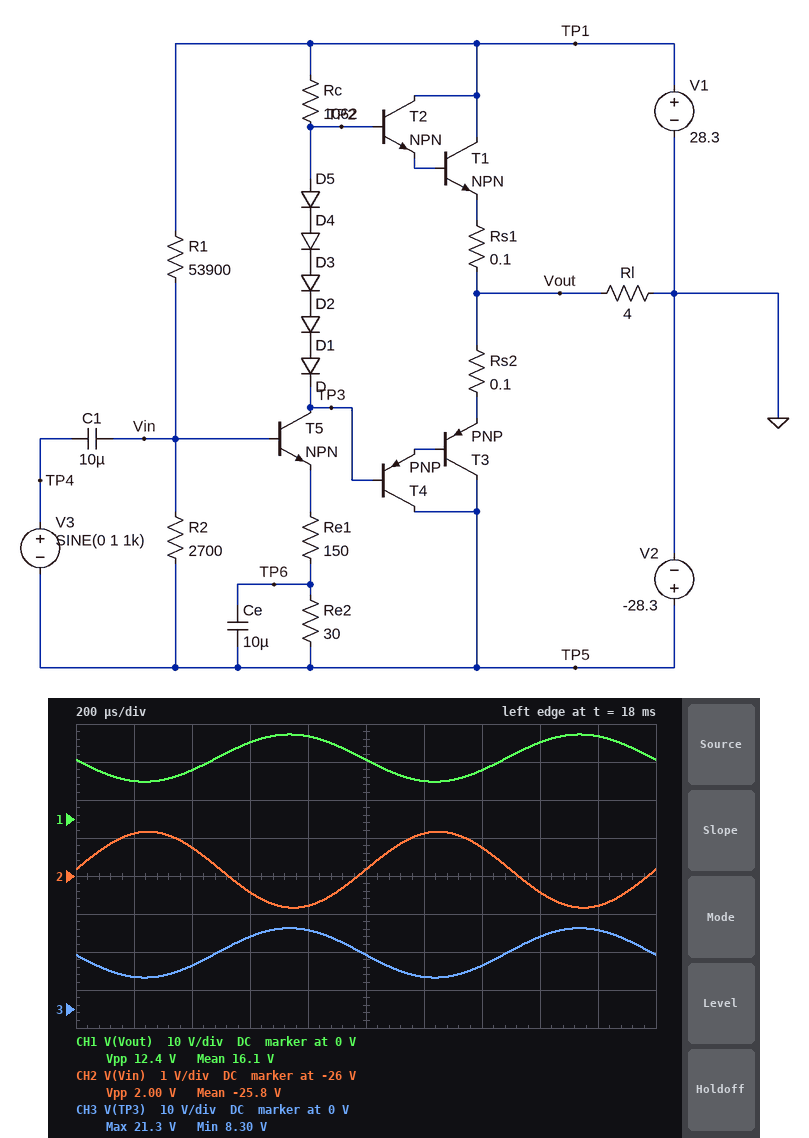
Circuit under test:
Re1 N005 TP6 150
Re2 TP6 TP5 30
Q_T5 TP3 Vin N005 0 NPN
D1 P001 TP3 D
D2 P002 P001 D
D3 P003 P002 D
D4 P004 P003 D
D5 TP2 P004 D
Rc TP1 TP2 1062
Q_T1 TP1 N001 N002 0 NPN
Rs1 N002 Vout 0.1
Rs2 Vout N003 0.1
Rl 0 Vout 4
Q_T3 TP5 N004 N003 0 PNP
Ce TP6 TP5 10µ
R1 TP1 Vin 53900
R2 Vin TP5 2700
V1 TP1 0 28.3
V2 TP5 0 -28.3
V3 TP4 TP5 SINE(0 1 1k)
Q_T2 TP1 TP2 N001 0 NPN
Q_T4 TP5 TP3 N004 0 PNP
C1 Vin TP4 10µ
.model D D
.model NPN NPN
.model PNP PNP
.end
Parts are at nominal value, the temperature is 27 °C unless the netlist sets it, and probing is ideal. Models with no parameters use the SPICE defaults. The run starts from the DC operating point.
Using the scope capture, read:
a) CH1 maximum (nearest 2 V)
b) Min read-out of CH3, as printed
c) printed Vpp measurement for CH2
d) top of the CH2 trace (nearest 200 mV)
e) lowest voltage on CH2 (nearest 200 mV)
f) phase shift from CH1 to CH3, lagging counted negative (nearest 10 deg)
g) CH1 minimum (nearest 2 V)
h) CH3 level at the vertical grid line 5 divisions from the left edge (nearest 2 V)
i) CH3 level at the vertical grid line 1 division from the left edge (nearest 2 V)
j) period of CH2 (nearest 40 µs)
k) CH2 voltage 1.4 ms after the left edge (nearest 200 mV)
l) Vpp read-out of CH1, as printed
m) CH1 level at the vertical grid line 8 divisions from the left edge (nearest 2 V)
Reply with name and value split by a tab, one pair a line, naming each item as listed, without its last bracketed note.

CH1 maximum	22 V
Min read-out of CH3, as printed	8.30 V
printed Vpp measurement for CH2	2.00 V
top of the CH2 trace	-24.8 V
lowest voltage on CH2	-26.8 V
phase shift from CH1 to CH3, lagging counted negative	0 deg
CH1 minimum	10 V
CH3 level at the vertical grid line 5 divisions from the left edge	14 V
CH3 level at the vertical grid line 1 division from the left edge	8 V
period of CH2	1.00 ms
CH2 voltage 1.4 ms after the left edge	-25.2 V
Vpp read-out of CH1, as printed	12.4 V
CH1 level at the vertical grid line 8 divisions from the left edge	20 V
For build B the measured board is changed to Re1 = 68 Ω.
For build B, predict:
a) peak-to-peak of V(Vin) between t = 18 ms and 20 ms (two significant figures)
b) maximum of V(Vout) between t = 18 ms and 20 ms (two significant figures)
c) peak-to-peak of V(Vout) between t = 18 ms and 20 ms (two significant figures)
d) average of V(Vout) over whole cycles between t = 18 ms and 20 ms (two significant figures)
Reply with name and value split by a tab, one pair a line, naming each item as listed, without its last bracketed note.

peak-to-peak of V(Vin) between t = 18 ms and 20 ms	2.0 V
maximum of V(Vout) between t = 18 ms and 20 ms	23 V
peak-to-peak of V(Vout) between t = 18 ms and 20 ms	26 V
average of V(Vout) over whole cycles between t = 18 ms and 20 ms	10 V
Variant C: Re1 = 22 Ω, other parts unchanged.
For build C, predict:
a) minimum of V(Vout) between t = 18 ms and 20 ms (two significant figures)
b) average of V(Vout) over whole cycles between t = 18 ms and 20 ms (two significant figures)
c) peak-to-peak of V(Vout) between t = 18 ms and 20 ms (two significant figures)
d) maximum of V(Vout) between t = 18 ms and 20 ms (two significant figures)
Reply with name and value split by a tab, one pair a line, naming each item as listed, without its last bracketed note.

minimum of V(Vout) between t = 18 ms and 20 ms	-24 V
average of V(Vout) over whole cycles between t = 18 ms and 20 ms	4.0 V
peak-to-peak of V(Vout) between t = 18 ms and 20 ms	49 V
maximum of V(Vout) between t = 18 ms and 20 ms	25 V
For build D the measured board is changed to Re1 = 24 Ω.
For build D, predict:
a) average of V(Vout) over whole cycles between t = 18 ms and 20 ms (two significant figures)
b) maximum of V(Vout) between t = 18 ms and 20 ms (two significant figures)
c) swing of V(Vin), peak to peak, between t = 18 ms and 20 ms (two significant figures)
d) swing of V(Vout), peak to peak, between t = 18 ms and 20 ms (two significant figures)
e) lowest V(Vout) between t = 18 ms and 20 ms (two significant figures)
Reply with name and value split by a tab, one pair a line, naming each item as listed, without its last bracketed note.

average of V(Vout) over whole cycles between t = 18 ms and 20 ms	3.4 V
maximum of V(Vout) between t = 18 ms and 20 ms	25 V
swing of V(Vin), peak to peak, between t = 18 ms and 20 ms	2.0 V
swing of V(Vout), peak to peak, between t = 18 ms and 20 ms	49 V
lowest V(Vout) between t = 18 ms and 20 ms	-24 V
